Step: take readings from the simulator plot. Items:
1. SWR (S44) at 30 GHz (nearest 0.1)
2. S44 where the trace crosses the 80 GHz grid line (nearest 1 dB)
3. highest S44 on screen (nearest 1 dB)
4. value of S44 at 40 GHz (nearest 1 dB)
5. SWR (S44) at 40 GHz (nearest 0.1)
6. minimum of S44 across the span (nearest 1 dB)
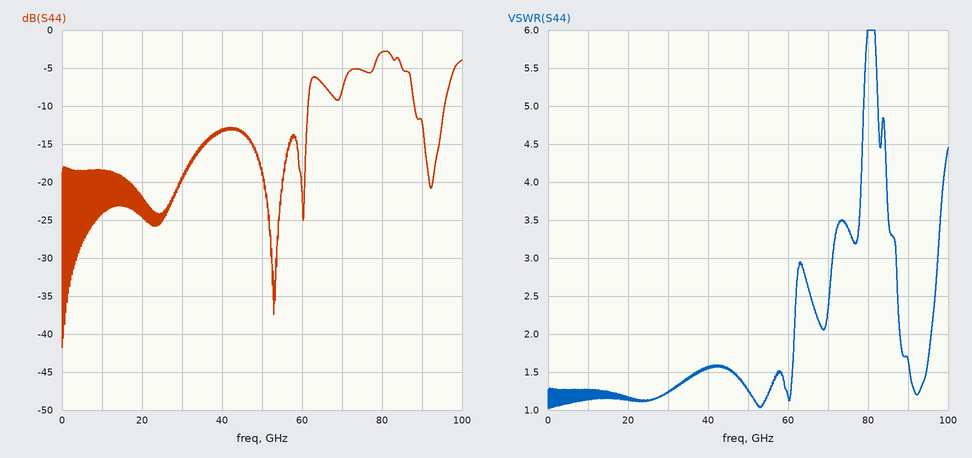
1.2
-3 dB
-3 dB
-13 dB
1.6
-42 dB
